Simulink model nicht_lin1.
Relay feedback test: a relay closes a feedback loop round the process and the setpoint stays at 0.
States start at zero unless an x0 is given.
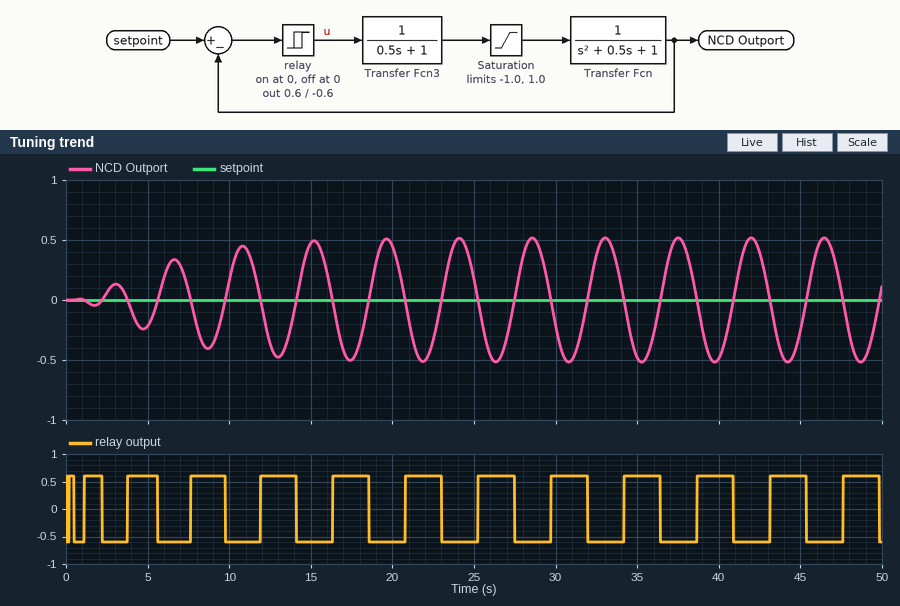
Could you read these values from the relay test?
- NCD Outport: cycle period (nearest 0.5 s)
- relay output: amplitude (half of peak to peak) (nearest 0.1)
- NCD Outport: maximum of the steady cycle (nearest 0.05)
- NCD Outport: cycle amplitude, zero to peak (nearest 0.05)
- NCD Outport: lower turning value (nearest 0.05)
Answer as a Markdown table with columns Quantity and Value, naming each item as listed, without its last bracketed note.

| Quantity | Value |
|---|---|
| NCD Outport: cycle period | 4.5 s |
| relay output: amplitude (half of peak to peak) | 0.6 |
| NCD Outport: maximum of the steady cycle | 0.50 |
| NCD Outport: cycle amplitude, zero to peak | 0.50 |
| NCD Outport: lower turning value | -0.50 |
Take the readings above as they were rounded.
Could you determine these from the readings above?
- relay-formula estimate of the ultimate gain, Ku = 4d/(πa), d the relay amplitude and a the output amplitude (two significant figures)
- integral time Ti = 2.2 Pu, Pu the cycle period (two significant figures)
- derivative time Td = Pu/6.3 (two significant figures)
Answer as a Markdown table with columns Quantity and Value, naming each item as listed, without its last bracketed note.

| Quantity | Value |
|---|---|
| relay-formula estimate of the ultimate gain, Ku = 4d/(πa), d the relay amplitude and a the output amplitude | 1.5 |
| integral time Ti = 2.2 Pu, Pu the cycle period | 9.9 s |
| derivative time Td = Pu/6.3 | 0.71 s |
